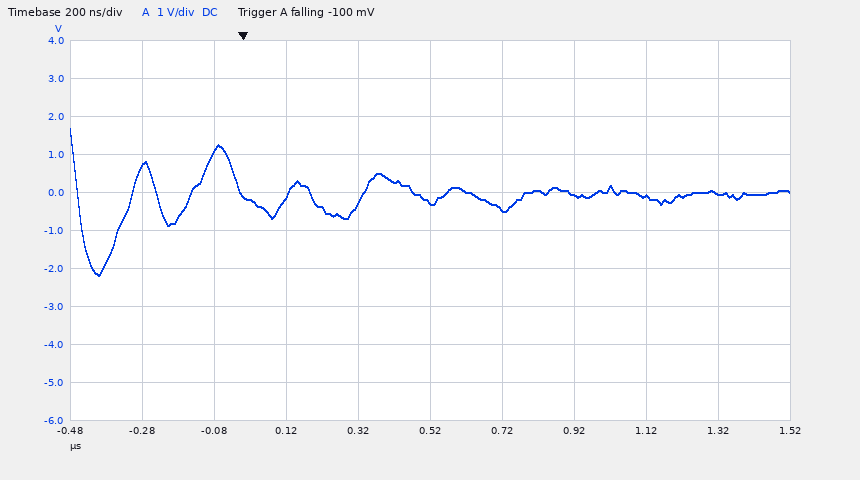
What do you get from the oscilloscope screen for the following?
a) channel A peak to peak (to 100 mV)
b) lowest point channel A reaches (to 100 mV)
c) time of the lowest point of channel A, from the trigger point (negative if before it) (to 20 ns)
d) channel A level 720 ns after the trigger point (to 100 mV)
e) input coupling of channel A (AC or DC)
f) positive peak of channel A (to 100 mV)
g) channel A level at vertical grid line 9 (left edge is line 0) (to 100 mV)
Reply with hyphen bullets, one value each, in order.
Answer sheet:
- 3.9 V
- -2.2 V
- -400 ns
- -400 mV
- DC
- 1.7 V
- 0.0 V
